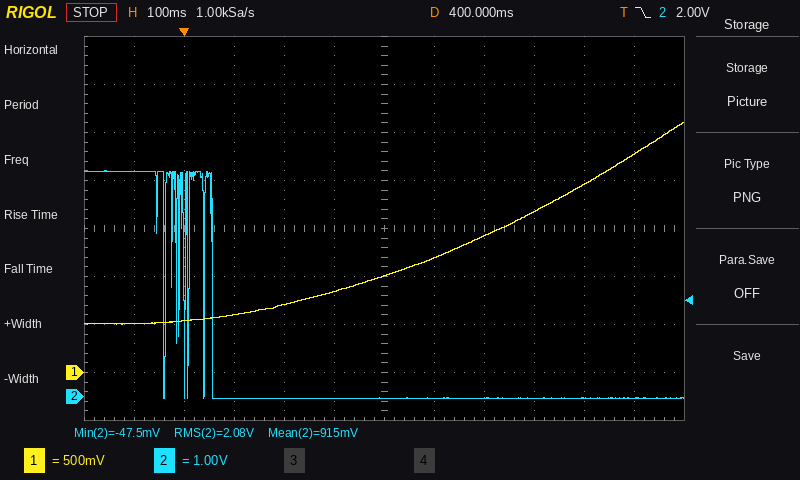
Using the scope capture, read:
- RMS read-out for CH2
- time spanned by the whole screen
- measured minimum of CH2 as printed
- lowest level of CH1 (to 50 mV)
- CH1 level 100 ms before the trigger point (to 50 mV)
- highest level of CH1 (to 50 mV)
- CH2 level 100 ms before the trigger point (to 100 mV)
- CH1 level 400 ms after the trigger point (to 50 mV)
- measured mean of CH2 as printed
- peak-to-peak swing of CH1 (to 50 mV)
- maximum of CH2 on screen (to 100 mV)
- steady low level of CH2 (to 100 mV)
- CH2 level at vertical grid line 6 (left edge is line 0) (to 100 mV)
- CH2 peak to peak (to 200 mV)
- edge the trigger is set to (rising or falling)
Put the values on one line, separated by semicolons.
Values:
2.08 V; 1.2 s; -47.5 mV; 500 mV; 500 mV; 2.60 V; 4.7 V; 1.00 V; 915 mV; 2.10 V; 4.7 V; 0.0 V; 0.0 V; 4.8 V; falling
